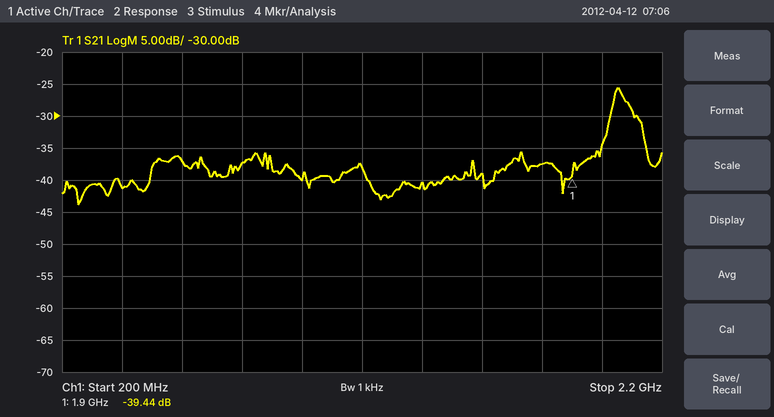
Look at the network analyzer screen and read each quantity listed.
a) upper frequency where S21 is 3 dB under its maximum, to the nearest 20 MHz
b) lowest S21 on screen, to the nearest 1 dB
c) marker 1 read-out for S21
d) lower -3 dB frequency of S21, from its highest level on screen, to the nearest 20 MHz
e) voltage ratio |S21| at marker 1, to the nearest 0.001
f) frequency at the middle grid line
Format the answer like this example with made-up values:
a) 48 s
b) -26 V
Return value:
a) 2.10 GHz
b) -44 dB
c) -39.44 dB
d) 2.04 GHz
e) 0.011
f) 1.2 GHz
